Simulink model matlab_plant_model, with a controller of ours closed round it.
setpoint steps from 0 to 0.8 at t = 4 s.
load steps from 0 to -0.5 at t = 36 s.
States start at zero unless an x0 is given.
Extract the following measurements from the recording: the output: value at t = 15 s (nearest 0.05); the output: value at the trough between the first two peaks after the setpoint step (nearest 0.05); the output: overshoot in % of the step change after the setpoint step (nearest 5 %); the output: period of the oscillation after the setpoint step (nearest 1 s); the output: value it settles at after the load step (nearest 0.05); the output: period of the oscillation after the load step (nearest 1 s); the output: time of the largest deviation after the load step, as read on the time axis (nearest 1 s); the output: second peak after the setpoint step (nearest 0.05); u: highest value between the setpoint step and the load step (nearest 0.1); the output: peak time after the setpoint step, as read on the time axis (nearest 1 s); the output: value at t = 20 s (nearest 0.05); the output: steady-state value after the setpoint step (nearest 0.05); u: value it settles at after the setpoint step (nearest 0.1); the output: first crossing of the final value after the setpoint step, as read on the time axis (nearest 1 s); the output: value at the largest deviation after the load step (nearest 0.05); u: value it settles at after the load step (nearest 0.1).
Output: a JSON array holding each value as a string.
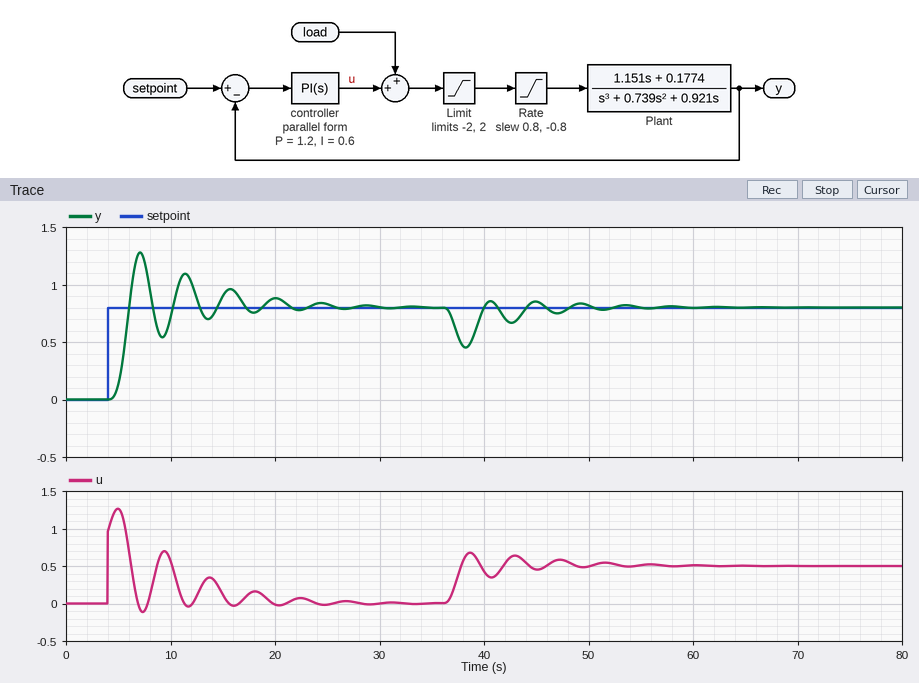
["0.90", "0.55", "60 %", "4 s", "0.80", "4 s", "38 s", "1.10", "1.3", "7 s", "0.90", "0.80", "0.0", "6 s", "0.45", "0.5"]
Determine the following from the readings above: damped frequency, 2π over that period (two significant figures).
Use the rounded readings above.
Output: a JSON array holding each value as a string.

["1.6 rad/s"]
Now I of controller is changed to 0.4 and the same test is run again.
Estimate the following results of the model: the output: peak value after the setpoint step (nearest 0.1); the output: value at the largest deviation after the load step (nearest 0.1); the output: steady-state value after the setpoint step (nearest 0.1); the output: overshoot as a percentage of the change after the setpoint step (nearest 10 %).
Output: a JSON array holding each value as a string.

["1.1", "0.4", "0.8", "40 %"]
